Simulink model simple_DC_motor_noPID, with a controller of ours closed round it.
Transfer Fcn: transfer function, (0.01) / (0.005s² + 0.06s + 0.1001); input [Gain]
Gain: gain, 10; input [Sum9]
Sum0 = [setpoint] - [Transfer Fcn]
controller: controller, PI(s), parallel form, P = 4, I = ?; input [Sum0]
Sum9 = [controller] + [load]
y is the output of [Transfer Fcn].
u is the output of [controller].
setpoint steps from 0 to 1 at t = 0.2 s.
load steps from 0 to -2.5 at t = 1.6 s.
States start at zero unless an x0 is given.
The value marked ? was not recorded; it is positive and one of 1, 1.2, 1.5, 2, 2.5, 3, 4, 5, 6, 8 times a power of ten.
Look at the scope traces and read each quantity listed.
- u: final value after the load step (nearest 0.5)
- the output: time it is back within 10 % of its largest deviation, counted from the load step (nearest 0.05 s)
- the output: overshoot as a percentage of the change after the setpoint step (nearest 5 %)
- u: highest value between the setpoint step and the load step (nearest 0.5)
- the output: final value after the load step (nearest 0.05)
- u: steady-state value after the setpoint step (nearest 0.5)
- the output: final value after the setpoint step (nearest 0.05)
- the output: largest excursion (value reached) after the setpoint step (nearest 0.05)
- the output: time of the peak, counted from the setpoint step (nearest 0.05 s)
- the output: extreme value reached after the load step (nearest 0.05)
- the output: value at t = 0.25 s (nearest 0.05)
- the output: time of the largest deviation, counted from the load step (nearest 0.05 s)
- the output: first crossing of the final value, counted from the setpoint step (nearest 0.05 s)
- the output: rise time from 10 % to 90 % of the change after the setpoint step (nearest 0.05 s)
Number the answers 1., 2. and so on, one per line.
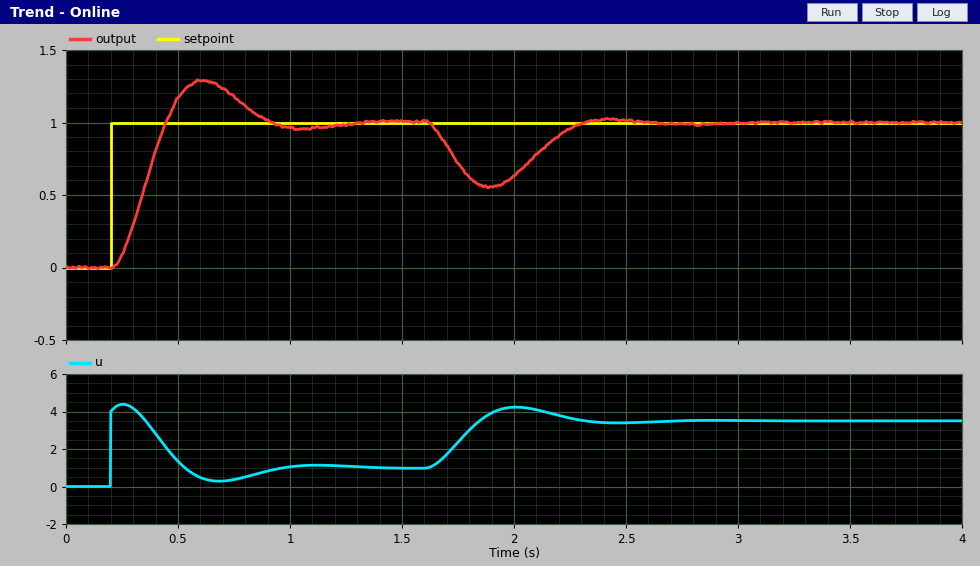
1. 3.5
2. 0.65 s
3. 30 %
4. 4.5
5. 1.00
6. 1.0
7. 1.00
8. 1.30
9. 0.40 s
10. 0.55
11. 0.10
12. 0.30 s
13. 0.25 s
14. 0.15 s
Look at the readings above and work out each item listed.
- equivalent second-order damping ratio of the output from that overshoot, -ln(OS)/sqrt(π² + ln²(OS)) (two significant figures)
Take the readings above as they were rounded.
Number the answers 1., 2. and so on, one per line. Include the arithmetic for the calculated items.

1. ln(0.3) = -1.204; 1.204 / sqrt(9.870 + 1.450) = 0.36
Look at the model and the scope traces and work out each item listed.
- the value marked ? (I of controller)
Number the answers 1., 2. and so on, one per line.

1. 15
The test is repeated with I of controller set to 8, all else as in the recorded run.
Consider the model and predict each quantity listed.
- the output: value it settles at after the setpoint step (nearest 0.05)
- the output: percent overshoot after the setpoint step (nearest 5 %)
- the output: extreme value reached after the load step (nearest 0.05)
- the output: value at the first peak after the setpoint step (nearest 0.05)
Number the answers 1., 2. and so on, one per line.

1. 1.00
2. 10 %
3. 0.50
4. 1.10
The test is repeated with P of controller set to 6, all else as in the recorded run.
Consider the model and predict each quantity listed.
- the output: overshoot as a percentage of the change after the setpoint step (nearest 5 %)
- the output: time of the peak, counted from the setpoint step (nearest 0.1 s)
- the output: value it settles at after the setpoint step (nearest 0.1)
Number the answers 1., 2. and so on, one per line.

1. 25 %
2. 0.3 s
3. 1.0
